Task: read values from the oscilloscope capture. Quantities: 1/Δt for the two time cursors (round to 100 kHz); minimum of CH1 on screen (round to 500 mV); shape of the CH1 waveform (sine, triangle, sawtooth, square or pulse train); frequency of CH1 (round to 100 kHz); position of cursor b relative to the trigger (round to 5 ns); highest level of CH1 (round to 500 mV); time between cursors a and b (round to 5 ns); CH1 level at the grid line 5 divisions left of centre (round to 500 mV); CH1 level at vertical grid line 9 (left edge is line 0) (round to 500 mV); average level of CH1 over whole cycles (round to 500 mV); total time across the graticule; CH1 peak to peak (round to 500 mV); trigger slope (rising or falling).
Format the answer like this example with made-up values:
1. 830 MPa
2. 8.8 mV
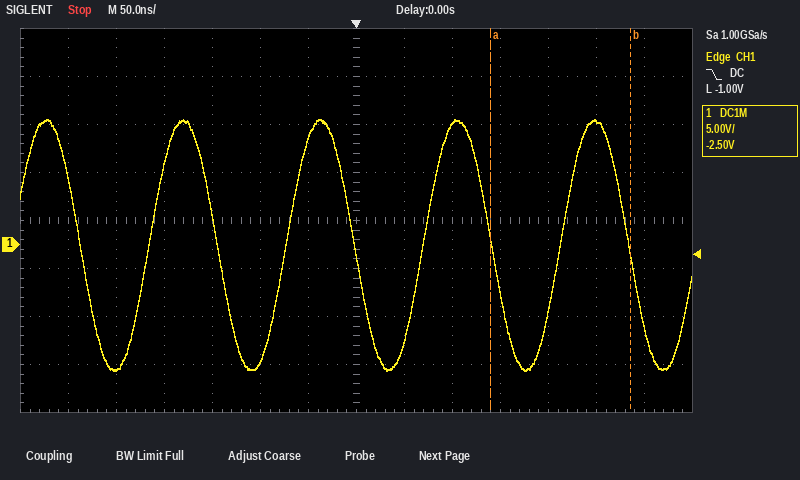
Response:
1. 6.9 MHz
2. -13.0 V
3. sine
4. 7.0 MHz
5. +285 ns
6. 13.0 V
7. 145 ns
8. -13.0 V
9. 12.5 V
10. 0.0 V
11. 700 ns
12. 26.0 V
13. falling
